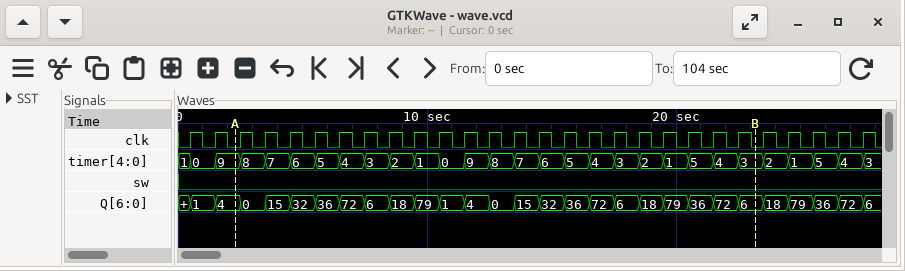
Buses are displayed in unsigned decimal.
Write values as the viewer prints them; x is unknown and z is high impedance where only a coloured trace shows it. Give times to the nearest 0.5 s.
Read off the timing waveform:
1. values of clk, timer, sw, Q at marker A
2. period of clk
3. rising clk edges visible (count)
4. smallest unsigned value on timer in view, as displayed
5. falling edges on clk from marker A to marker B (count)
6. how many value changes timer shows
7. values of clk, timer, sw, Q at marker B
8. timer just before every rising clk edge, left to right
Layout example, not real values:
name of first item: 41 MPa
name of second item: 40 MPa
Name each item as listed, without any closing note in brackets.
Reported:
values of clk, timer, sw, Q at marker A: clk=0, timer=9, sw=0, Q=4
period of clk: 1 s
rising clk edges visible: 28
smallest unsigned value on timer in view, as displayed: 0
falling edges on clk from marker A to marker B: 21
how many value changes timer shows: 28
values of clk, timer, sw, Q at marker B: clk=0, timer=3, sw=0, Q=6
timer just before every rising clk edge, left to right: 1, 0, 9, 8, 7, 6, 5, 4, 3, 2, 1, 0, 9, 8, 7, 6, 5, 4, 3, 2, 1, 5, 4, 3, 2, 1, 5, 4
